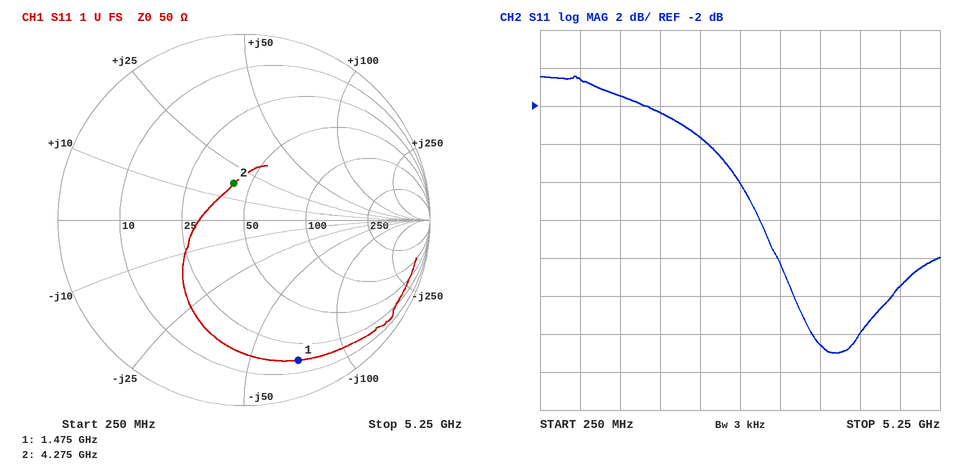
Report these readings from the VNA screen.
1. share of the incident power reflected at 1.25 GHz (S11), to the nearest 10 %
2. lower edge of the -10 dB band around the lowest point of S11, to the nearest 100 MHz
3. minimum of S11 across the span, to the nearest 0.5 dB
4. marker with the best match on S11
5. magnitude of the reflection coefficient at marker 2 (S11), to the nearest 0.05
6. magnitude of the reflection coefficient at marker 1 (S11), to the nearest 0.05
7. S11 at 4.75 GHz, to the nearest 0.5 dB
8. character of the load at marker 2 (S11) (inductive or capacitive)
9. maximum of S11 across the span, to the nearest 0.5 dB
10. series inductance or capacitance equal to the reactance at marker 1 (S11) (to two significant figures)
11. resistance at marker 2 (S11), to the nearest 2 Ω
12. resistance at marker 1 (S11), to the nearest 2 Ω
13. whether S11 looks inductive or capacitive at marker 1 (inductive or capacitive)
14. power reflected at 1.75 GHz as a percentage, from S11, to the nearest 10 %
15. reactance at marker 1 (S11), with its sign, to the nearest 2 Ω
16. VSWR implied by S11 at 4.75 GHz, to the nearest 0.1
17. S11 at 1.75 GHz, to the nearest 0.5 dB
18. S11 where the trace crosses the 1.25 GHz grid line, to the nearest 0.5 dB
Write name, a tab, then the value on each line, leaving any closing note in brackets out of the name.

share of the incident power reflected at 1.25 GHz (S11), to the nearest 10 %	70 %
lower edge of the -10 dB band around the lowest point of S11, to the nearest 100 MHz	3.2 GHz
minimum of S11 across the span, to the nearest 0.5 dB	-15.0 dB
marker with the best match on S11	marker 2
magnitude of the reflection coefficient at marker 2 (S11), to the nearest 0.05	0.20
magnitude of the reflection coefficient at marker 1 (S11), to the nearest 0.05	0.80
S11 at 4.75 GHz, to the nearest 0.5 dB	-11.5 dB
character of the load at marker 2 (S11)	inductive
maximum of S11 across the span, to the nearest 0.5 dB	-0.5 dB
series inductance or capacitance equal to the reactance at marker 1 (S11)	1.5 pF
resistance at marker 2 (S11), to the nearest 2 Ω	42 Ω
resistance at marker 1 (S11), to the nearest 2 Ω	16 Ω
whether S11 looks inductive or capacitive at marker 1	capacitive
power reflected at 1.75 GHz as a percentage, from S11, to the nearest 10 %	60 %
reactance at marker 1 (S11), with its sign, to the nearest 2 Ω	-70 Ω
VSWR implied by S11 at 4.75 GHz, to the nearest 0.1	1.7
S11 at 1.75 GHz, to the nearest 0.5 dB	-2.5 dB
S11 where the trace crosses the 1.25 GHz grid line, to the nearest 0.5 dB	-1.5 dB
